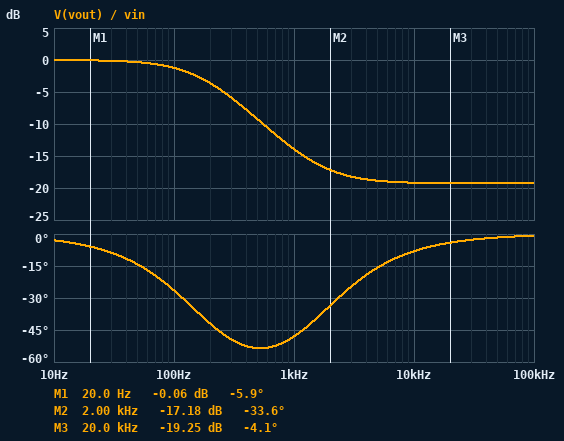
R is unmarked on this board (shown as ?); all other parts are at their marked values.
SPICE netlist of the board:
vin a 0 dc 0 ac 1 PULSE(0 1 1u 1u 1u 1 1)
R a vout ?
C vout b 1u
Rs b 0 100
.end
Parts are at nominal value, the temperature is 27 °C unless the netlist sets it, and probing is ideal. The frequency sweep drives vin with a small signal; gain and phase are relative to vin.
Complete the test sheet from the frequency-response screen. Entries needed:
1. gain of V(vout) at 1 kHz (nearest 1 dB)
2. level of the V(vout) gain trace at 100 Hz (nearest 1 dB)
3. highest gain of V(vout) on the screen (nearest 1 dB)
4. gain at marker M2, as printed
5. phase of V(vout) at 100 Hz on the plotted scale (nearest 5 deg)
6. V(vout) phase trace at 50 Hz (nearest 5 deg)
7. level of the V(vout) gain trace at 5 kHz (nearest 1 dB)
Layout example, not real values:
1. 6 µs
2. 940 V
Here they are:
1. -14 dB
2. -1 dB
3. 0 dB
4. -17.18 dB
5. -25 deg
6. -15 deg
7. -19 dB
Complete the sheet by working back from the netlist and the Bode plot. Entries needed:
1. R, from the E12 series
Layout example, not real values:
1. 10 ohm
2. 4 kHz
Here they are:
1. 820 Ω
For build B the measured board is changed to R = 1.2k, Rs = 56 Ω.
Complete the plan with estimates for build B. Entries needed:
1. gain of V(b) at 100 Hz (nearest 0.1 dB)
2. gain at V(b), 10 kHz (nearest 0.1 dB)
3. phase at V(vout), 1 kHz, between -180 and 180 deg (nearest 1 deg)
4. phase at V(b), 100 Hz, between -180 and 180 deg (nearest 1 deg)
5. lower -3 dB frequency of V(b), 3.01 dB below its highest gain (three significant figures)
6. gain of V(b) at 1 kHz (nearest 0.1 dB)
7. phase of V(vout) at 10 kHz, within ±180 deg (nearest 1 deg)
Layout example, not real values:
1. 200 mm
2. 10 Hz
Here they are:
1. -31.2 dB
2. -27.0 dB
3. -63 deg
4. 52 deg
5. 127 Hz
6. -27.1 dB
7. -15 deg
